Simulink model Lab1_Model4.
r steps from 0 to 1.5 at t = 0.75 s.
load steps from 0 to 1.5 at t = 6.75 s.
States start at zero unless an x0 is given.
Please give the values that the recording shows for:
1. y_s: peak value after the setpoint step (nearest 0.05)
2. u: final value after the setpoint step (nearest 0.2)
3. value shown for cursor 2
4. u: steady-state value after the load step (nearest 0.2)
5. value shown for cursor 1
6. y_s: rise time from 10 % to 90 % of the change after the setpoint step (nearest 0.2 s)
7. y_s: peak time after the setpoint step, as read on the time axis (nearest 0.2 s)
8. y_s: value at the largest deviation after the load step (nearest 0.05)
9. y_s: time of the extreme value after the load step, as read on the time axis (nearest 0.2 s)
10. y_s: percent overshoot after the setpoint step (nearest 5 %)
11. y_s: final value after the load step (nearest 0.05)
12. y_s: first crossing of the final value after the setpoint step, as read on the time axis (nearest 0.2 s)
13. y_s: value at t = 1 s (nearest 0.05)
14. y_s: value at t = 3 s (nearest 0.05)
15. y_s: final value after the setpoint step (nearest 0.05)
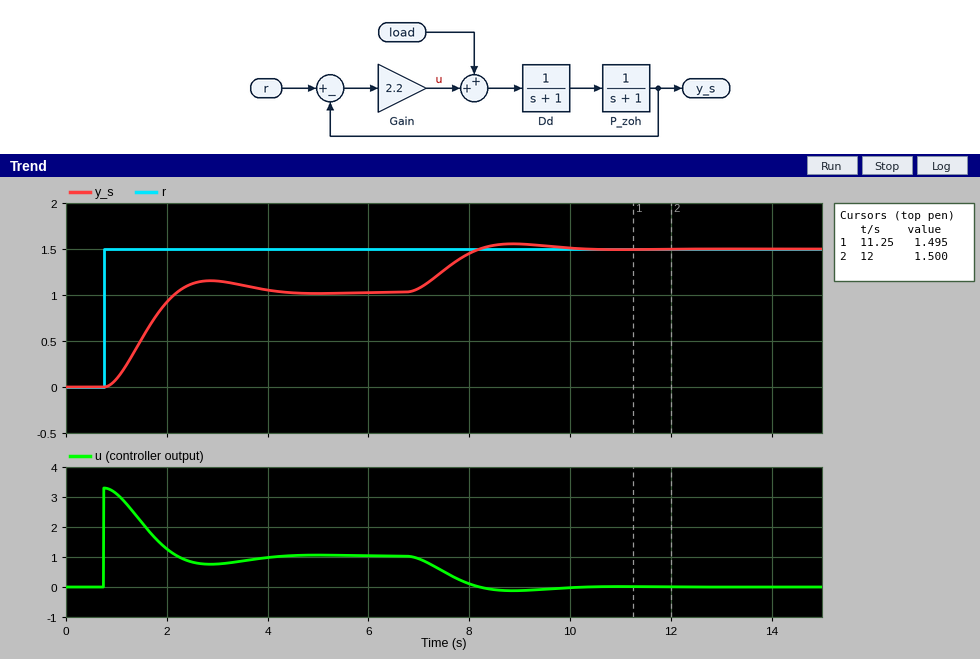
1.15
1.0
1.500
0.0
1.495
1.0 s
2.8 s
1.55
8.8 s
10 %
1.50
2.2 s
0.10
1.15
1.05
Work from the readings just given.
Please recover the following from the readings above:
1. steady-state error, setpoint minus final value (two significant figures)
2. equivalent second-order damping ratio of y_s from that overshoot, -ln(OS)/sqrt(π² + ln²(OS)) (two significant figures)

0.45
0.59
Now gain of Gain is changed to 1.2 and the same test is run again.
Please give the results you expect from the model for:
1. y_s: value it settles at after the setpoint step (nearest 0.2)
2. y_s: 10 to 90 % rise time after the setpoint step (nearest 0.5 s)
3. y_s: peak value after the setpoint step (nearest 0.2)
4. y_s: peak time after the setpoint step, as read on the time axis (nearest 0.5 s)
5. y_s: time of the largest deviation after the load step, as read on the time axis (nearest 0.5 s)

0.8
1.5 s
0.8
3.5 s
9.5 s
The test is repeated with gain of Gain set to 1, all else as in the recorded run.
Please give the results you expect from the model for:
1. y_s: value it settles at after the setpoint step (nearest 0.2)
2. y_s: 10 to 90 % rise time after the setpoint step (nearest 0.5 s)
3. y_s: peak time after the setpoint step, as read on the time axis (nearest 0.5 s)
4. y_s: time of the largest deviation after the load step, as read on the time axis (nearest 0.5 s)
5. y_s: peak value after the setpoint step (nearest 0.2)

0.8
1.5 s
4.0 s
10.0 s
0.8
